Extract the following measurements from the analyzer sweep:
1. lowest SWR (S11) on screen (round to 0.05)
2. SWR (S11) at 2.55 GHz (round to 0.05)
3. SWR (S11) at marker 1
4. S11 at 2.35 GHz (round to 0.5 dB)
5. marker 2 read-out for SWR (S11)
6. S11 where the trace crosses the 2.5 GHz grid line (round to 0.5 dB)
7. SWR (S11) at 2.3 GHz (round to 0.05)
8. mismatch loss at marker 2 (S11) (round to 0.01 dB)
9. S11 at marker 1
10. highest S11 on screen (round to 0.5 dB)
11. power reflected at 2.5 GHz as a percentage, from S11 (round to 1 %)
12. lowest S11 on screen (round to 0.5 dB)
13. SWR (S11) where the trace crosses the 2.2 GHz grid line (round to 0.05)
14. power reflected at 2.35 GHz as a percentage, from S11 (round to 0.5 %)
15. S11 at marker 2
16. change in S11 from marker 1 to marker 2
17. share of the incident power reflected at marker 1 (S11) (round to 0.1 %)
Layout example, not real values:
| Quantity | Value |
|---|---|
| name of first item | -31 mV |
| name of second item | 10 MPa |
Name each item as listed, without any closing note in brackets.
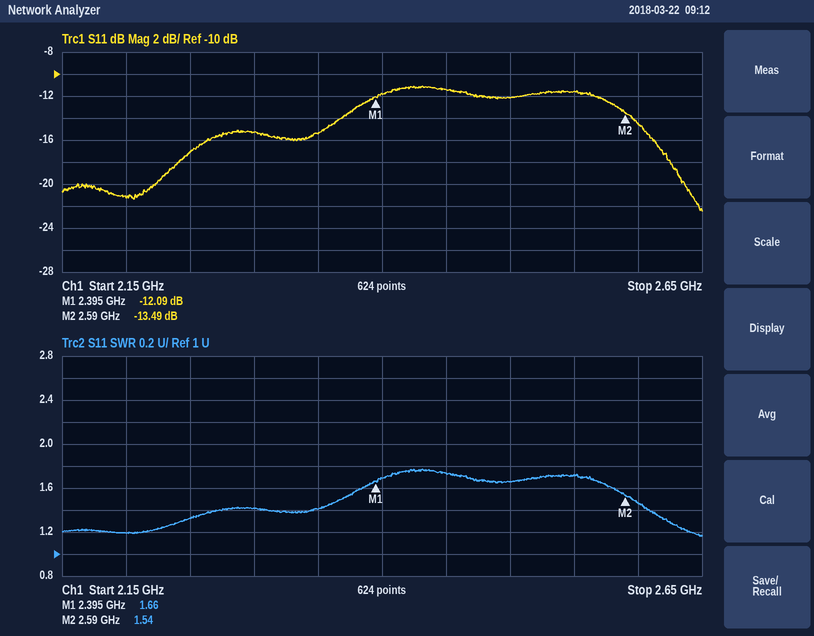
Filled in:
| Quantity | Value |
|---|---|
| lowest SWR (S11) on screen | 1.15 |
| SWR (S11) at 2.55 GHz | 1.70 |
| SWR (S11) at marker 1 | 1.66 |
| S11 at 2.35 GHz | -15.5 dB |
| marker 2 read-out for SWR | 1.54 |
| S11 where the trace crosses the 2.5 GHz grid line | -12.0 dB |
| SWR (S11) at 2.3 GHz | 1.40 |
| mismatch loss at marker 2 (S11) | 0.20 dB |
| S11 at marker 1 | -12.09 dB |
| highest S11 on screen | -11.0 dB |
| power reflected at 2.5 GHz as a percentage, from S11 | 6 % |
| lowest S11 on screen | -22.5 dB |
| SWR (S11) where the trace crosses the 2.2 GHz grid line | 1.20 |
| power reflected at 2.35 GHz as a percentage, from S11 | 3.0 % |
| S11 at marker 2 | -13.49 dB |
| change in S11 from marker 1 to marker 2 | -1.40 dB |
| share of the incident power reflected at marker 1 (S11) | 6.2 % |
